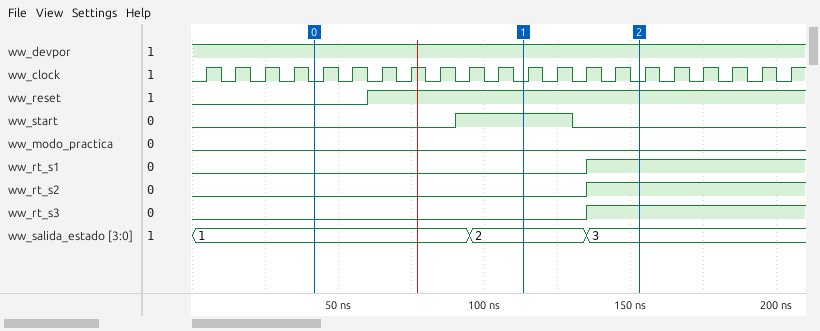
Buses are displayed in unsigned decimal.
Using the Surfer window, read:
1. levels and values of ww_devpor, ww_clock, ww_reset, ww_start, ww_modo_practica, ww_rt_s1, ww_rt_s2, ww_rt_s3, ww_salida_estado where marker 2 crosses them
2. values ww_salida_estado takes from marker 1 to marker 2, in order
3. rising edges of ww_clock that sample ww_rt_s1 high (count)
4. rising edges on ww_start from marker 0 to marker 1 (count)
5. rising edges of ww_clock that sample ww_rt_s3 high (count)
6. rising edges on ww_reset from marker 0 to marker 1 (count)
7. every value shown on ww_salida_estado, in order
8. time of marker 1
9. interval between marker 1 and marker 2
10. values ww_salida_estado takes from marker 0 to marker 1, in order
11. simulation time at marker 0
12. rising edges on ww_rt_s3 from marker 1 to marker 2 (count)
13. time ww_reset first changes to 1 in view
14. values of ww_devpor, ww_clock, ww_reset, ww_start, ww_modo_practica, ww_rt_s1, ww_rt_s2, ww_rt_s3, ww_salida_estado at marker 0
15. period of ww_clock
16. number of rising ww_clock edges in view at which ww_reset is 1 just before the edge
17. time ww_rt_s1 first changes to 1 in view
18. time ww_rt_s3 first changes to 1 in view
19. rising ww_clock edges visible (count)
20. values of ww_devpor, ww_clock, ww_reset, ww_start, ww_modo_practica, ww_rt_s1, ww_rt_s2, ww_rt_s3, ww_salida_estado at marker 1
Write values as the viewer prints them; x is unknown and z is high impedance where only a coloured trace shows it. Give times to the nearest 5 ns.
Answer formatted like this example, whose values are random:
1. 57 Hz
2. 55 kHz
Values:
1. ww_devpor=1, ww_clock=0, ww_reset=1, ww_start=0, ww_modo_practica=0, ww_rt_s1=1, ww_rt_s2=1, ww_rt_s3=1, ww_salida_estado=3
2. 2, 3
3. 7
4. 1
5. 7
6. 1
7. 1, 2, 3
8. 115 ns
9. 40 ns
10. 1, 2
11. 40 ns
12. 1
13. 60 ns
14. ww_devpor=1, ww_clock=0, ww_reset=0, ww_start=0, ww_modo_practica=0, ww_rt_s1=0, ww_rt_s2=0, ww_rt_s3=0, ww_salida_estado=1
15. 10 ns
16. 15
17. 135 ns
18. 135 ns
19. 21
20. ww_devpor=1, ww_clock=0, ww_reset=1, ww_start=1, ww_modo_practica=0, ww_rt_s1=0, ww_rt_s2=0, ww_rt_s3=0, ww_salida_estado=2
